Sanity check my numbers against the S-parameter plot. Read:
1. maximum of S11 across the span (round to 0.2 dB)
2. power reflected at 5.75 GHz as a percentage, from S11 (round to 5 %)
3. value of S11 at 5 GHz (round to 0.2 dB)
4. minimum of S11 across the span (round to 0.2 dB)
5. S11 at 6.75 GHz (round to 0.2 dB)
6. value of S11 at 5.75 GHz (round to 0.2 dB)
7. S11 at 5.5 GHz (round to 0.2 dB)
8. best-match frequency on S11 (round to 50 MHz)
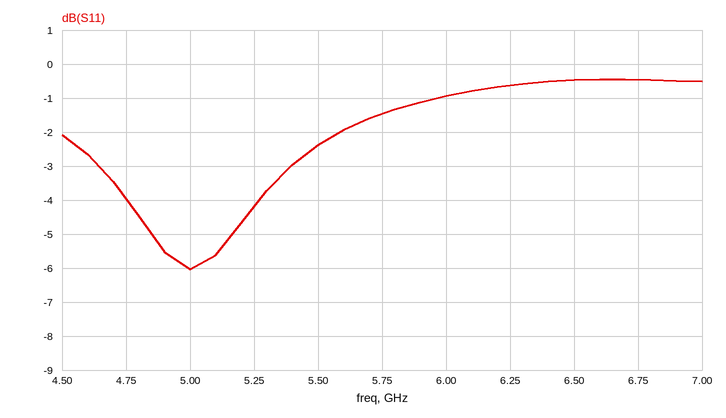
-0.4 dB
70 %
-6.0 dB
-6.0 dB
-0.4 dB
-1.4 dB
-2.4 dB
5.00 GHz
